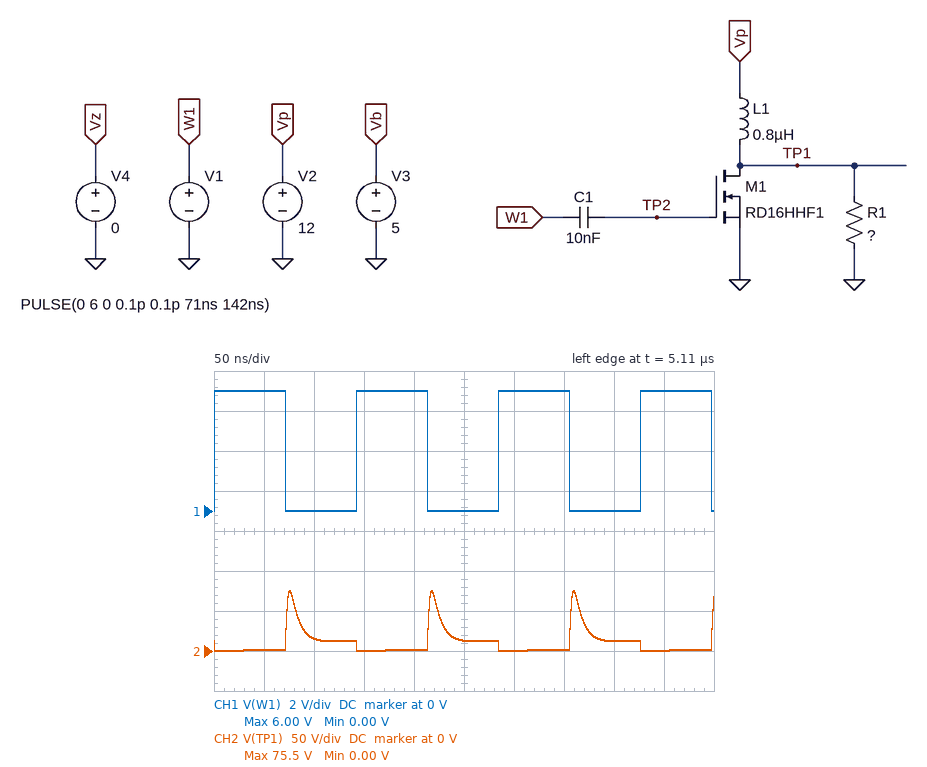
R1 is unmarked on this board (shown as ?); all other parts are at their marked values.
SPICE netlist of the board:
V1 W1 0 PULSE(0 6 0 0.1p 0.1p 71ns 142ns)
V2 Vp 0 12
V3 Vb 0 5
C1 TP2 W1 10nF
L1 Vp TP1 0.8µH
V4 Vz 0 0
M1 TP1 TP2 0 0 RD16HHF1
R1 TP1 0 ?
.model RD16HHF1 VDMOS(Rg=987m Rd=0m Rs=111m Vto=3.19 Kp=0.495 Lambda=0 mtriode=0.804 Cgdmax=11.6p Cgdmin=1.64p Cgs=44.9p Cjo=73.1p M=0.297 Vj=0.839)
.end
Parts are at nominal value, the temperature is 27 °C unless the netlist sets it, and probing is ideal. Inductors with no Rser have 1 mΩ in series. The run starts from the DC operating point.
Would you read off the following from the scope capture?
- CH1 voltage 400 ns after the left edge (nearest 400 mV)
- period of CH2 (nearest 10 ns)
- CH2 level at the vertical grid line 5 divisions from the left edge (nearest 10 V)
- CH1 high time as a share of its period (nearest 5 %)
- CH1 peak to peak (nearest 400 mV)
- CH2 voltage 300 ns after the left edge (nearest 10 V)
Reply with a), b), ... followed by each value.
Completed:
a) 0 V
b) 140 ns
c) 10 V
d) 50 %
e) 6.0 V
f) 0 V
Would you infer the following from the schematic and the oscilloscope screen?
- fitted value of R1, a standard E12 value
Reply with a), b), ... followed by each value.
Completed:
a) 82 Ω
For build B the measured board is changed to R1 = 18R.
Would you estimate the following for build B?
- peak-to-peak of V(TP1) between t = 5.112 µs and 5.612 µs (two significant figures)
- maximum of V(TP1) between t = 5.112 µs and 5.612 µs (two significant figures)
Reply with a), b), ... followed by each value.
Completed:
a) 31 V
b) 32 V
